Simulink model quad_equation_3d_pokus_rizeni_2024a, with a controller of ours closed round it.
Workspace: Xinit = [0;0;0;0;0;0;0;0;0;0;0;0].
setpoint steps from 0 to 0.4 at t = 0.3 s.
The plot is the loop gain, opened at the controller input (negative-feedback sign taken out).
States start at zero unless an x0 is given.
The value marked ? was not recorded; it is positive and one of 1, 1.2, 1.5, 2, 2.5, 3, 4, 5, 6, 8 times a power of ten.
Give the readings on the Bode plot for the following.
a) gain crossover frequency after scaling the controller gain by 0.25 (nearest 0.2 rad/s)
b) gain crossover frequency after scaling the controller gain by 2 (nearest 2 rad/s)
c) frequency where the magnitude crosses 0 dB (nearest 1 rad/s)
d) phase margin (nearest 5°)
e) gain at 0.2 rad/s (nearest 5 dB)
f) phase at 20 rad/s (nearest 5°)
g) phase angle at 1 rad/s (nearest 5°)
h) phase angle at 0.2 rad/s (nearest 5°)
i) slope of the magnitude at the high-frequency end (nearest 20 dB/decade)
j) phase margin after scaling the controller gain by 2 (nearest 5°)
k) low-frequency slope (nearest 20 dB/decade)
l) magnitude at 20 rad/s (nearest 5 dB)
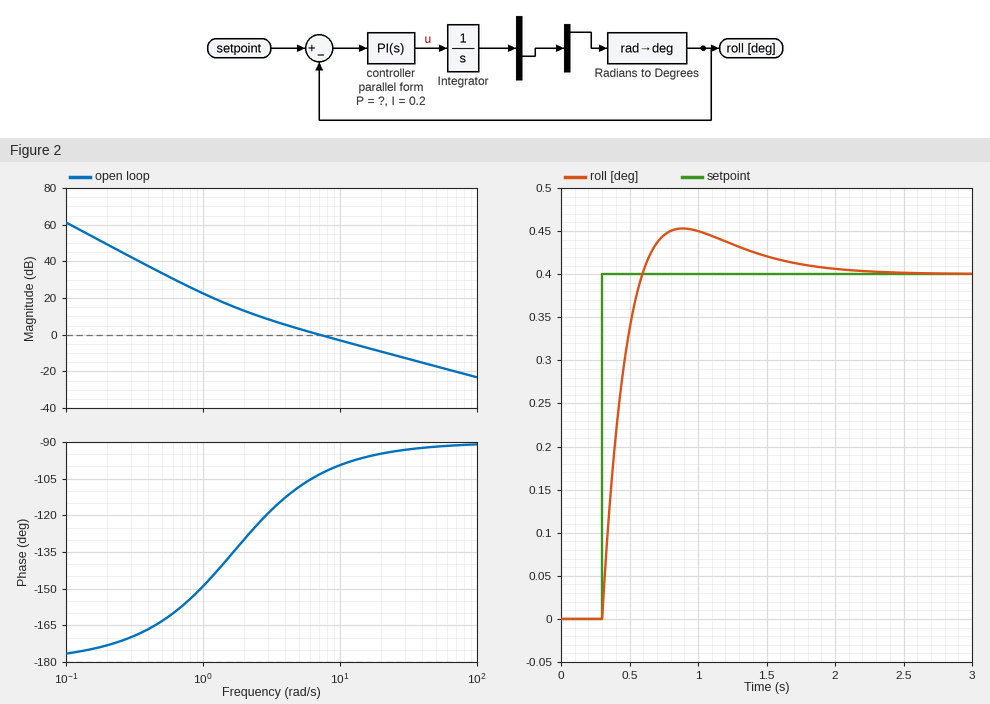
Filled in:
2.2 rad/s
14 rad/s
7 rad/s
75°
50 dB
-95°
-150°
-175°
-20 dB/decade
85°
-40 dB/decade
-10 dB
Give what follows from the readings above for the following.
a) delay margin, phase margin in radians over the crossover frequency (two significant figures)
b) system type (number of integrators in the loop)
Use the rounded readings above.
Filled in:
0.19 s
2
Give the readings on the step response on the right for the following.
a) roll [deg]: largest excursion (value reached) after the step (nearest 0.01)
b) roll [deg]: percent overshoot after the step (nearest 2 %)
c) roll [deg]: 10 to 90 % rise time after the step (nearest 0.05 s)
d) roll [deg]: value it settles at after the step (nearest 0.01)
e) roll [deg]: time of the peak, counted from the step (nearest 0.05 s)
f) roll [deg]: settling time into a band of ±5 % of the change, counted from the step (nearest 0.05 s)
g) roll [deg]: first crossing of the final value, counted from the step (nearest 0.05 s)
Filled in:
0.45
14 %
0.20 s
0.40
0.60 s
1.20 s
0.30 s
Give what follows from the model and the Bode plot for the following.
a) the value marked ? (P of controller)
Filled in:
0.12
